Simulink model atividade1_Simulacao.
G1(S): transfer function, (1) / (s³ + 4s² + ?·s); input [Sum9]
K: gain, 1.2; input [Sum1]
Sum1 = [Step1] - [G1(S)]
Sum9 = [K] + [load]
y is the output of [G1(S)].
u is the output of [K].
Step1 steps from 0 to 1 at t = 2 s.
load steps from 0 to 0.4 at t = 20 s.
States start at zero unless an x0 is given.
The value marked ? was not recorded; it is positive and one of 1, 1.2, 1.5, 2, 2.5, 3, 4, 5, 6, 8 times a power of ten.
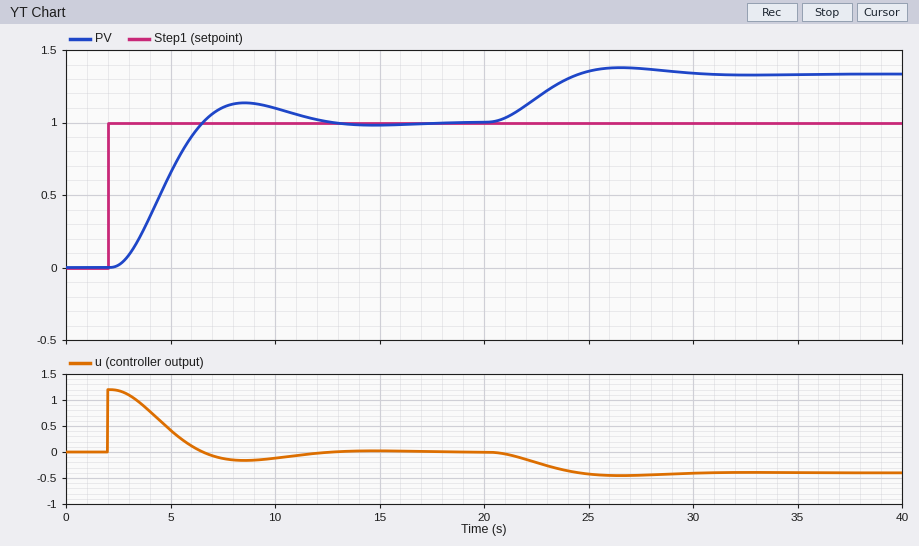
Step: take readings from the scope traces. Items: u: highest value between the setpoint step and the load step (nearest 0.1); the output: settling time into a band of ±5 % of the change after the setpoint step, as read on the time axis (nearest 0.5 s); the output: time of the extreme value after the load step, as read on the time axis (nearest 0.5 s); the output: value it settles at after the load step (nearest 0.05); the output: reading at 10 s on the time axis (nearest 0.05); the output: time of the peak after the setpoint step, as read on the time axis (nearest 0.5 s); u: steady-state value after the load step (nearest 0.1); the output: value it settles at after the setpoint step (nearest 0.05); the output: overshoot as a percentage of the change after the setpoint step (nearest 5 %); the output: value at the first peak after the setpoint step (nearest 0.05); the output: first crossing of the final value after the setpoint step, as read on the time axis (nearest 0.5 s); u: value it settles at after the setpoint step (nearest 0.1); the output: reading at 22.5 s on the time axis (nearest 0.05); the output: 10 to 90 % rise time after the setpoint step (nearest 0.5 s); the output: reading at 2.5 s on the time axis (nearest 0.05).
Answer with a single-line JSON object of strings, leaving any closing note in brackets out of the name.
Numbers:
{"u: highest value between the setpoint step and the load step": "1.2", "the output: settling time into a band of ±5 % of the change after the setpoint step, as read on the time axis": "11.0 s", "the output: time of the extreme value after the load step, as read on the time axis": "26.5 s", "the output: value it settles at after the load step": "1.35", "the output: reading at 10 s on the time axis": "1.10", "the output: time of the peak after the setpoint step, as read on the time axis": "8.5 s", "u: steady-state value after the load step": "-0.4", "the output: value it settles at after the setpoint step": "1.00", "the output: overshoot as a percentage of the change after the setpoint step": "15 %", "the output: value at the first peak after the setpoint step": "1.15", "the output: first crossing of the final value after the setpoint step, as read on the time axis": "6.5 s", "u: value it settles at after the setpoint step": "0.0", "the output: reading at 22.5 s on the time axis": "1.15", "the output: 10 to 90 % rise time after the setpoint step": "3.0 s", "the output: reading at 2.5 s on the time axis": "0.00"}
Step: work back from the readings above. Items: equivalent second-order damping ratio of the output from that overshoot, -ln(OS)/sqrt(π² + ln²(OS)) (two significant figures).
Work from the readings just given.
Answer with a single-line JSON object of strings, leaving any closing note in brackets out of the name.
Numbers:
{"equivalent second-order damping ratio of the output from that overshoot, -ln(OS)/sqrt(π² + ln²(OS))": "0.52"}
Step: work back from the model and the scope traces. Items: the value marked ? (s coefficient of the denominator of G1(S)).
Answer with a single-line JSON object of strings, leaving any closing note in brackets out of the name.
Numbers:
{"the value marked ? (s coefficient of the denominator of G1(S))": "2.5"}
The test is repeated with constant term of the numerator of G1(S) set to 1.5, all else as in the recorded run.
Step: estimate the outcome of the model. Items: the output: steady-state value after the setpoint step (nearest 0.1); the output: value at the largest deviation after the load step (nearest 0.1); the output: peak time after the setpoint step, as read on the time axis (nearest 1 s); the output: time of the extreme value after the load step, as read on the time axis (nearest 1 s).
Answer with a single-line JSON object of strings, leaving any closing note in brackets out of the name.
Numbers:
{"the output: steady-state value after the setpoint step": "1.0", "the output: value at the largest deviation after the load step": "1.4", "the output: peak time after the setpoint step, as read on the time axis": "7 s", "the output: time of the extreme value after the load step, as read on the time axis": "25 s"}
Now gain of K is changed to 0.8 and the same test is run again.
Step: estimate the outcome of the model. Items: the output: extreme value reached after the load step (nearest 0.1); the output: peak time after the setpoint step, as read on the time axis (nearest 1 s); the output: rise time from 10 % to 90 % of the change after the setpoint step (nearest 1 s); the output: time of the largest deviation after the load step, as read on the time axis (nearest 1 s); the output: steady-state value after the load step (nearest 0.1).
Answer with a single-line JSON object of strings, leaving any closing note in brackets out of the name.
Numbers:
{"the output: extreme value reached after the load step": "1.5", "the output: peak time after the setpoint step, as read on the time axis": "11 s", "the output: rise time from 10 % to 90 % of the change after the setpoint step": "4 s", "the output: time of the largest deviation after the load step, as read on the time axis": "29 s", "the output: steady-state value after the load step": "1.5"}
